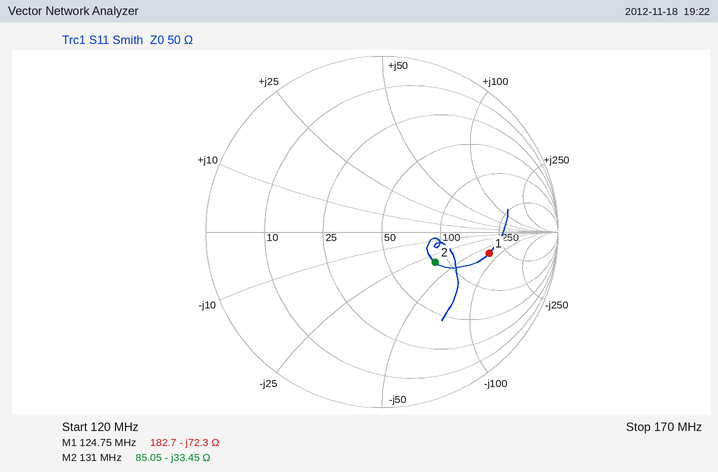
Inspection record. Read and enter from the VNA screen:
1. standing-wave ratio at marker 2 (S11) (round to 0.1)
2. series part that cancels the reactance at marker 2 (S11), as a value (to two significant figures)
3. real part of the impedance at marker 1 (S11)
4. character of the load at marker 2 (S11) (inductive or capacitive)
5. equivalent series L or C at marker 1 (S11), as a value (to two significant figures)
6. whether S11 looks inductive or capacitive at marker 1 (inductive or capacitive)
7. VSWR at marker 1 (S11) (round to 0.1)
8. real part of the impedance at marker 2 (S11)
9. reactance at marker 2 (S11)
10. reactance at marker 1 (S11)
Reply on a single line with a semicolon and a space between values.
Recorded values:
2.1; 41 nH; 182.7 Ω; capacitive; 18 pF; capacitive; 4.3; 85.05 Ω; -33.45 Ω; -72.3 Ω
